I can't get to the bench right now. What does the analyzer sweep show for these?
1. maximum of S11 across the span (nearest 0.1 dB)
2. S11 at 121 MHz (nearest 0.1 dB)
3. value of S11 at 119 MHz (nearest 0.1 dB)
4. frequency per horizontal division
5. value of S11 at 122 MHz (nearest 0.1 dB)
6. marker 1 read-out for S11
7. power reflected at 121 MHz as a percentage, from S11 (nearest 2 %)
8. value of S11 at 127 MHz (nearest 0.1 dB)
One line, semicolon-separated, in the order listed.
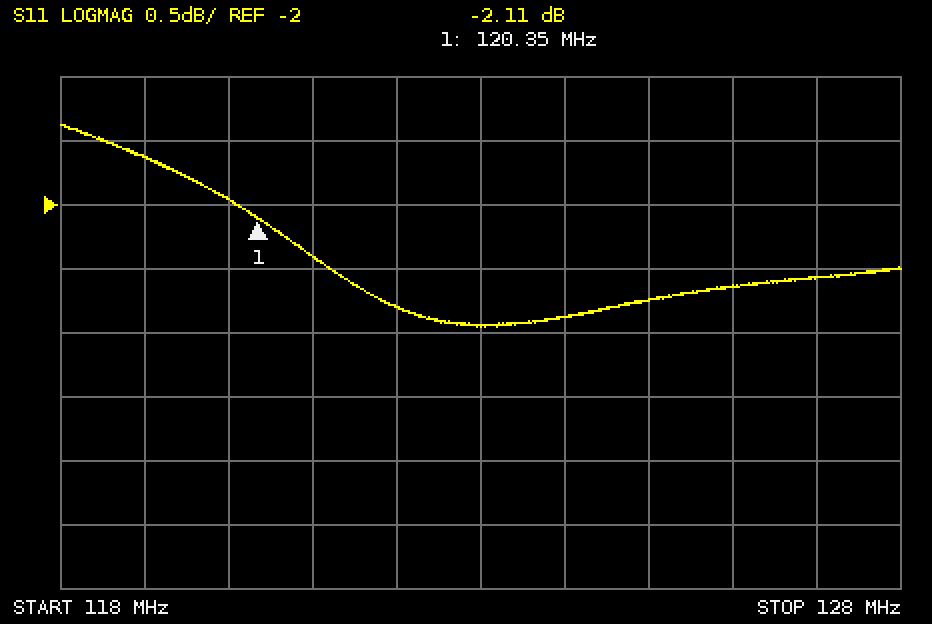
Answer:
-1.4 dB; -2.4 dB; -1.6 dB; 1 MHz; -2.8 dB; -2.11 dB; 58 %; -2.6 dB
